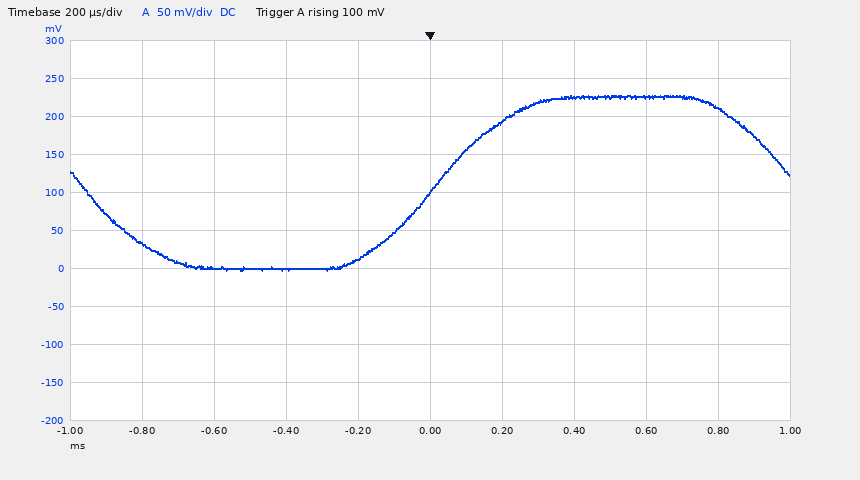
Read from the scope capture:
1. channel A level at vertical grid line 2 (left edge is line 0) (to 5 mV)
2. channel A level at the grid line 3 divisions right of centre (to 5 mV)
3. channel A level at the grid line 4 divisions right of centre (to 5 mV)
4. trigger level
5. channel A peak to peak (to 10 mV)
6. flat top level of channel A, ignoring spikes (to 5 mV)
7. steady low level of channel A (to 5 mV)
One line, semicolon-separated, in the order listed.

0 mV; 225 mV; 210 mV; 100 mV; 230 mV; 225 mV; 0 mV
